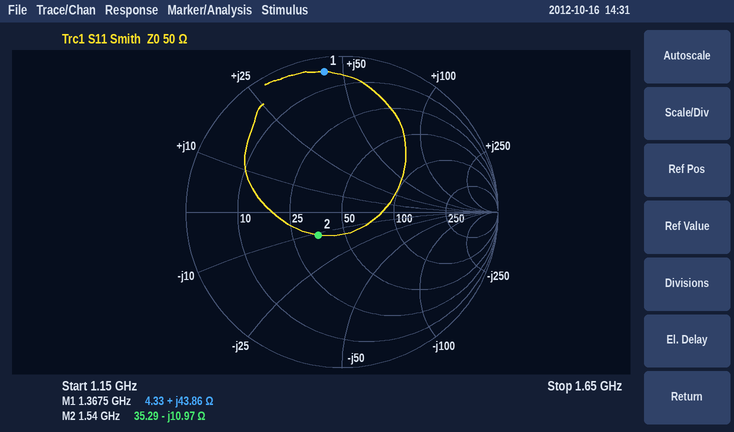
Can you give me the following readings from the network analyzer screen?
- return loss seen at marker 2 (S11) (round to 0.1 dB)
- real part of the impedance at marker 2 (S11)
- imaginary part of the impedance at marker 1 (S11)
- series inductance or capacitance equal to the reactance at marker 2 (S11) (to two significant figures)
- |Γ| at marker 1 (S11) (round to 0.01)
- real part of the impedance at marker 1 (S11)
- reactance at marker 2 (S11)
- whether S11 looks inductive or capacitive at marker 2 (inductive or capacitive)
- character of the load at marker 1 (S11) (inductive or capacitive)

13.4 dB
35.29 Ω
+43.86 Ω
9.4 pF
0.91
4.33 Ω
-10.97 Ω
capacitive
inductive
